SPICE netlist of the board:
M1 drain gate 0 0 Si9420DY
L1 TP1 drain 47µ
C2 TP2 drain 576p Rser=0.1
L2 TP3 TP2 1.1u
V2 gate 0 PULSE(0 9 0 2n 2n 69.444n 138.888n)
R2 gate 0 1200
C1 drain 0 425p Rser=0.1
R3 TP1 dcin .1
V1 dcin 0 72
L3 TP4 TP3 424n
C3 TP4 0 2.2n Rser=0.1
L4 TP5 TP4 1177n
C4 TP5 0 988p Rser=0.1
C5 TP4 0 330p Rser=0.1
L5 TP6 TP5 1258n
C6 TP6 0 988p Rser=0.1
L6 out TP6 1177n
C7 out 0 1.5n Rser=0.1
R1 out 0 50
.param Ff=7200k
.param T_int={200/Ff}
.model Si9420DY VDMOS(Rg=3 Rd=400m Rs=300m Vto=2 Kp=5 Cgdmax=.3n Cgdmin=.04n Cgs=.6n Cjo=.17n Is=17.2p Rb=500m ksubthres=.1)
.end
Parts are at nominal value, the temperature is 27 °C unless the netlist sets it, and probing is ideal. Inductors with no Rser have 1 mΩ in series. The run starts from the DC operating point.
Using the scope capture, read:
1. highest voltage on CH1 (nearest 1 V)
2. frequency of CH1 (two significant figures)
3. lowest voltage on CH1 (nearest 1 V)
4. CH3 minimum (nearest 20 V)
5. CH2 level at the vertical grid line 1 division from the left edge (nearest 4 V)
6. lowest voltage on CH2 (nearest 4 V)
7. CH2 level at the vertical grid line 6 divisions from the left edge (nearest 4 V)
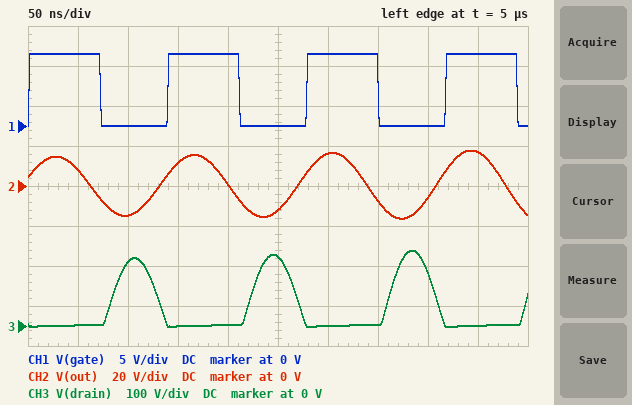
9 V
7.2 MHz
0 V
0 V
8 V
-16 V
16 V
